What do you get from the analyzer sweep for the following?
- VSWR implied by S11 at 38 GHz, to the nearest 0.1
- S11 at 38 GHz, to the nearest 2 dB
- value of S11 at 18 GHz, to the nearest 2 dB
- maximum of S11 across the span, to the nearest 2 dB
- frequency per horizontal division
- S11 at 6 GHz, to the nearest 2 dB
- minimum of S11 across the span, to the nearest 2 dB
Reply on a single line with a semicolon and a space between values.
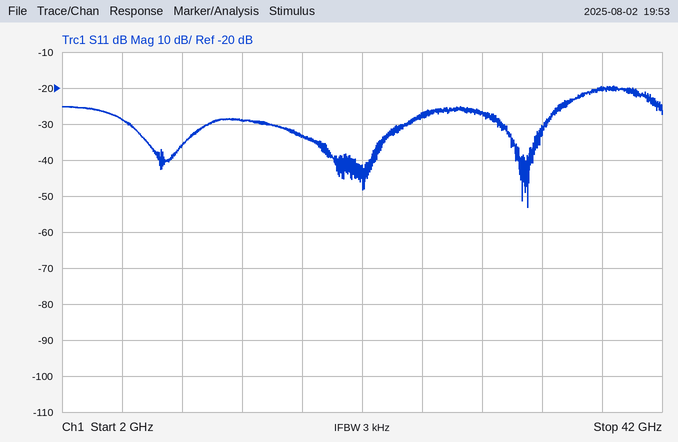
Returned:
1.2; -20 dB; -34 dB; -20 dB; 4 GHz; -28 dB; -54 dB
